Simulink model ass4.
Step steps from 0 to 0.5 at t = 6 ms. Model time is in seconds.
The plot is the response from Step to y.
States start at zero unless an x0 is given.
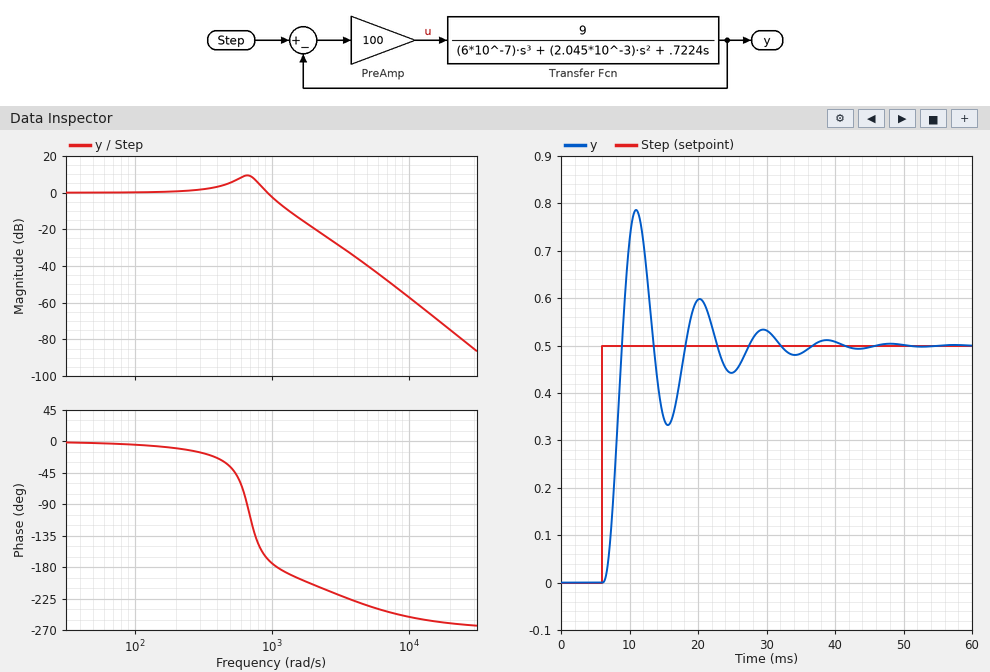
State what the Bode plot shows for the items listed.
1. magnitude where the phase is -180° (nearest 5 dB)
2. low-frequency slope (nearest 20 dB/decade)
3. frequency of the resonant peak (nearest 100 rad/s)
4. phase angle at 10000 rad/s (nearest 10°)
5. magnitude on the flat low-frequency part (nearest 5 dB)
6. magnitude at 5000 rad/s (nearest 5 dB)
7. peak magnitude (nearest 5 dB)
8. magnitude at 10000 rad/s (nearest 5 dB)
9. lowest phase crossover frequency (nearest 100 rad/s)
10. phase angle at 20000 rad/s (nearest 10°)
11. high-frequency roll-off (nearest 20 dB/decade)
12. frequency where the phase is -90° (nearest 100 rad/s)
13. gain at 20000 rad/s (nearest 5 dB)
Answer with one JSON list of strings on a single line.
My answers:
["-5 dB", "0 dB/decade", "700 rad/s", "-250°", "0 dB", "-40 dB", "10 dB", "-55 dB", "1100 rad/s", "-260°", "-60 dB/decade", "700 rad/s", "-75 dB"]
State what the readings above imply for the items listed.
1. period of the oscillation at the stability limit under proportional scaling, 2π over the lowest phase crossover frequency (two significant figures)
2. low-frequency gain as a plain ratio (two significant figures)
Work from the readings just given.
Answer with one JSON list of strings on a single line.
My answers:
["0.0057 s", "1.0"]
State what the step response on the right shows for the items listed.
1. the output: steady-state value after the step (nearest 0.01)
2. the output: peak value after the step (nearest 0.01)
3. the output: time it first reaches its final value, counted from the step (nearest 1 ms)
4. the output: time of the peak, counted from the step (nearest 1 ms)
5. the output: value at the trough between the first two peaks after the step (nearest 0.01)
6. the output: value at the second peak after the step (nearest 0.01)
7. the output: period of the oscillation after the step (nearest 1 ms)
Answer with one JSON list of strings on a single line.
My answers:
["0.50", "0.79", "3 ms", "5 ms", "0.33", "0.60", "9 ms"]
